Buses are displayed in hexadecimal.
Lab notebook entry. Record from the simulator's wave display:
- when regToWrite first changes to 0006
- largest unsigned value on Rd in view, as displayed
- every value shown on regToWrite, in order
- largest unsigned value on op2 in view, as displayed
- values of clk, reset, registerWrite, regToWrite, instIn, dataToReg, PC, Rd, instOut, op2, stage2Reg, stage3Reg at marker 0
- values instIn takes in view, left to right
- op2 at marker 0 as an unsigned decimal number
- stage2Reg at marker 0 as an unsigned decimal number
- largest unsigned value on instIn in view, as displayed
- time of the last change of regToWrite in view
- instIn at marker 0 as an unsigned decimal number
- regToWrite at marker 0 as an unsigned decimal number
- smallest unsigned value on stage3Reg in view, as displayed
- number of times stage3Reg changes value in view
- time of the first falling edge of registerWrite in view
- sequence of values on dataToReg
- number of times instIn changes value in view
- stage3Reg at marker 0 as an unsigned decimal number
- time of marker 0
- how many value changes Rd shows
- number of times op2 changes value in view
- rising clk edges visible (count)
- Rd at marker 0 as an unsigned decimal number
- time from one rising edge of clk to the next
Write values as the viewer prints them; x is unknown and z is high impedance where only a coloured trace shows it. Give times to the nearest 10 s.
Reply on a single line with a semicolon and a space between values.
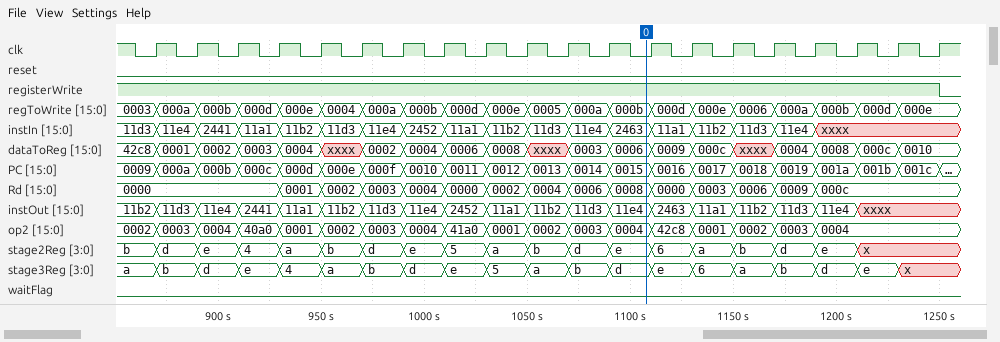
1150 s; 000c; 0003, 000a, 000b, 000d, 000e, 0004, 000a, 000b, 000d, 000e, 0005, 000a, 000b, 000d, 000e, 0006, 000a, 000b, 000d, 000e; 42c8; clk=0, reset=0, registerWrite=1, regToWrite=000b, instIn=2463, dataToReg=0006, PC=0015, Rd=0008, instOut=11e4, op2=0004, stage2Reg=e, stage3Reg=d; 11d3, 11e4, 2441, 11a1, 11b2, 11d3, 11e4, 2452, 11a1, 11b2, 11d3, 11e4, 2463, 11a1, 11b2, 11d3, 11e4, xxxx; 4; 14; 2463; 1230 s; 9315; 11; 4; 19; 1250 s; 42c8, 0001, 0002, 0003, 0004, xxxx, 0002, 0004, 0006, 0008, xxxx, 0003, 0006, 0009, 000c, xxxx, 0004, 0008, 000c, 0010; 17; 13; 1110 s; 14; 17; 20; 8; 20 s
